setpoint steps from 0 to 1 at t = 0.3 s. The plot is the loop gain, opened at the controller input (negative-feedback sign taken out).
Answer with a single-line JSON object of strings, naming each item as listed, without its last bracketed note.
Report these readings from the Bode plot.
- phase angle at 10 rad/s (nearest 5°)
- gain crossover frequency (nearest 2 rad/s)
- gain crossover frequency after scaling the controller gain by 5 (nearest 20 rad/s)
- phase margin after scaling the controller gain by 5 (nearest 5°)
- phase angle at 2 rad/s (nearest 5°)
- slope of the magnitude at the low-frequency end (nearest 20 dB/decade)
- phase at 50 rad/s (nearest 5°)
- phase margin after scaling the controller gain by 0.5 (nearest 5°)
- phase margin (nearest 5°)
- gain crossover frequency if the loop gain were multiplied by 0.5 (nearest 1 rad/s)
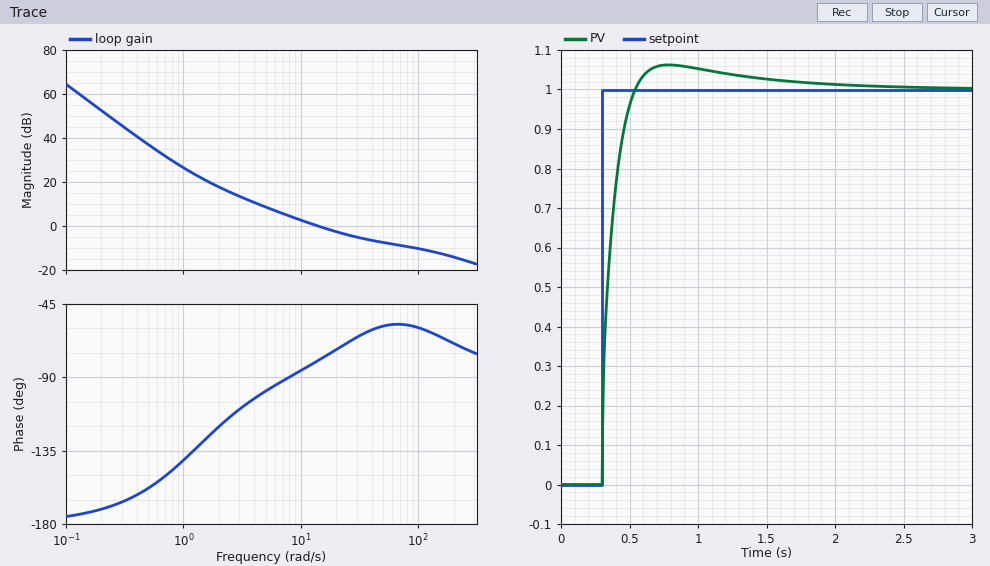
{"phase angle at 10 rad/s": "-85°", "gain crossover frequency": "14 rad/s", "gain crossover frequency after scaling the controller gain by 5": "200 rad/s", "phase margin after scaling the controller gain by 5": "110°", "phase angle at 2 rad/s": "-120°", "slope of the magnitude at the low-frequency end": "-40 dB/decade", "phase at 50 rad/s": "-60°", "phase margin after scaling the controller gain by 0.5": "85°", "phase margin": "100°", "gain crossover frequency if the loop gain were multiplied by 0.5": "7 rad/s"}
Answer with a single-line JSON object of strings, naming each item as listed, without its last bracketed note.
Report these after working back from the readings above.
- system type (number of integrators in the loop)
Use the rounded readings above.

{"system type": "2"}
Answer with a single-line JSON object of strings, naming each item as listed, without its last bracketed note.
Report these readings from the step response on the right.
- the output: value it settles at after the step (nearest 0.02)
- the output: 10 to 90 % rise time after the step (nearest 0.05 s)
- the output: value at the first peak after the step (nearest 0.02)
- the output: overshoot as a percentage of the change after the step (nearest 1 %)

{"the output: value it settles at after the step": "1.00", "the output: 10 to 90 % rise time after the step": "0.15 s", "the output: value at the first peak after the step": "1.06", "the output: overshoot as a percentage of the change after the step": "6 %"}
